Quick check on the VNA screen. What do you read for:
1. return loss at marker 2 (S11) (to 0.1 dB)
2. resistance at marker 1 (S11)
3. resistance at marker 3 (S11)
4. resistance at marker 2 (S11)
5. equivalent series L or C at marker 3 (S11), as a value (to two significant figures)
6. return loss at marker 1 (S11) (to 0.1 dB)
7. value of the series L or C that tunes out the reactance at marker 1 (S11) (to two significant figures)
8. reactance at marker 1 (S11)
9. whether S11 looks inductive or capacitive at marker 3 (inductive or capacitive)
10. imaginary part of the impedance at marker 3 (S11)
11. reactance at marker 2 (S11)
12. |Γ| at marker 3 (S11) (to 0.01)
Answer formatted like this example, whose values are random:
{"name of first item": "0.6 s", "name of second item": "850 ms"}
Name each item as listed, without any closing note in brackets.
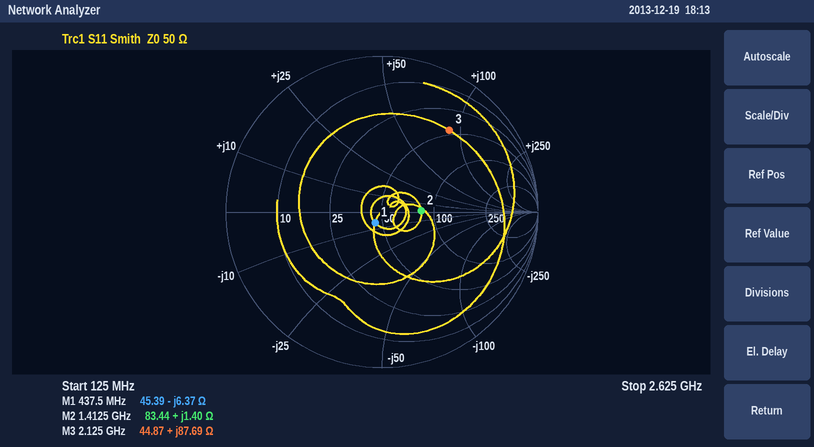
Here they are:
{"return loss at marker 2 (S11)": "12.0 dB", "resistance at marker 1": "45.39 Ω", "resistance at marker 3": "44.87 Ω", "resistance at marker 2": "83.44 Ω", "equivalent series L or C at marker 3 (S11), as a value": "6.6 nH", "return loss at marker 1 (S11)": "21.7 dB", "value of the series L or C that tunes out the reactance at marker 1 (S11)": "2.3 nH", "reactance at marker 1": "-6.37 Ω", "whether S11 looks inductive or capacitive at marker 3": "inductive", "imaginary part of the impedance at marker 3": "+87.69 Ω", "reactance at marker 2": "+1.40 Ω", "|Γ| at marker 3 (S11)": "0.68"}
